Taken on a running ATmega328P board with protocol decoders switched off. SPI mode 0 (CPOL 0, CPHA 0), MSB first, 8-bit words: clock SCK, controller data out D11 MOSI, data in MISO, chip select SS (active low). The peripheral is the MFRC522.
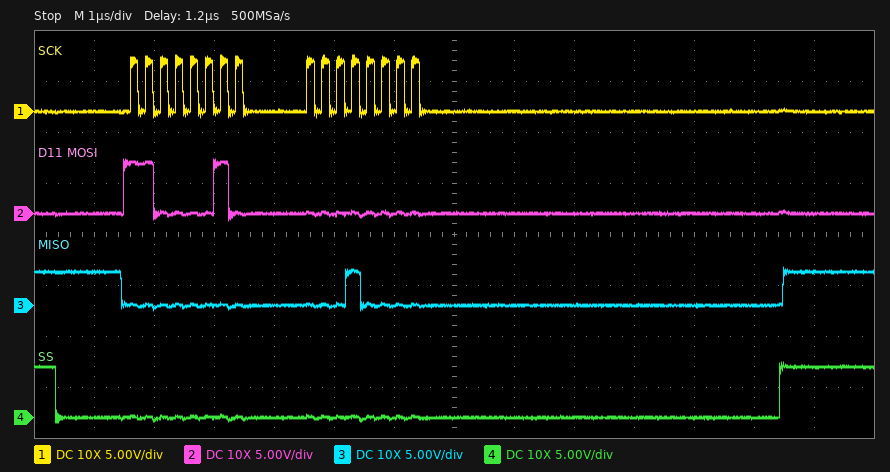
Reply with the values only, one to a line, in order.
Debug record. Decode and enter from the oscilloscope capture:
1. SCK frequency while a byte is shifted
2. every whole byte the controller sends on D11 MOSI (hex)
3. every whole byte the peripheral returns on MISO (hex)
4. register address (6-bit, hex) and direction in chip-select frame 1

4 MHz
C2 00
00 10
0x21 read
